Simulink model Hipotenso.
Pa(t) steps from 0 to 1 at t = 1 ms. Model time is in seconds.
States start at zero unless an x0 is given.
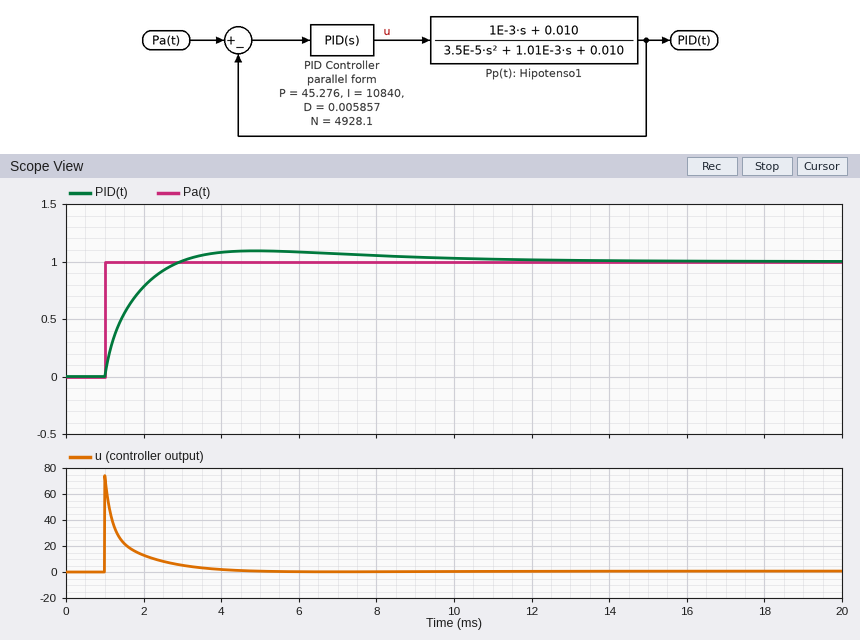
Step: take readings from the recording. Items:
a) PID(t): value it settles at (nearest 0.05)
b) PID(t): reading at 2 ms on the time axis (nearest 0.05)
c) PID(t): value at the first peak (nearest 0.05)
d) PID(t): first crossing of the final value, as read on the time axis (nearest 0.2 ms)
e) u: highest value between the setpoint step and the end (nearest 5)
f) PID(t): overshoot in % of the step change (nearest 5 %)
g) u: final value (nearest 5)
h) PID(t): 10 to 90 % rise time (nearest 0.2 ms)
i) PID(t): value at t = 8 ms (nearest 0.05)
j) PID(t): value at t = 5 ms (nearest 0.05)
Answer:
1.00
0.80
1.10
3.0 ms
75
10 %
0
1.4 ms
1.05
1.10
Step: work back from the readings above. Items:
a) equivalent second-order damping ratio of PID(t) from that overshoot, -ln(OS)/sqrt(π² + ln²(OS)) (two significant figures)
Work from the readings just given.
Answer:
0.59
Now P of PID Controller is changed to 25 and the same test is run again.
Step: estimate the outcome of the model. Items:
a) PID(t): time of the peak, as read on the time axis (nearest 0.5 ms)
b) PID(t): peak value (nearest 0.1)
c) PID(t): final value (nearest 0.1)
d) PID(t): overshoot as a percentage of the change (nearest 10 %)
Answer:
5.5 ms
1.2
1.0
20 %
